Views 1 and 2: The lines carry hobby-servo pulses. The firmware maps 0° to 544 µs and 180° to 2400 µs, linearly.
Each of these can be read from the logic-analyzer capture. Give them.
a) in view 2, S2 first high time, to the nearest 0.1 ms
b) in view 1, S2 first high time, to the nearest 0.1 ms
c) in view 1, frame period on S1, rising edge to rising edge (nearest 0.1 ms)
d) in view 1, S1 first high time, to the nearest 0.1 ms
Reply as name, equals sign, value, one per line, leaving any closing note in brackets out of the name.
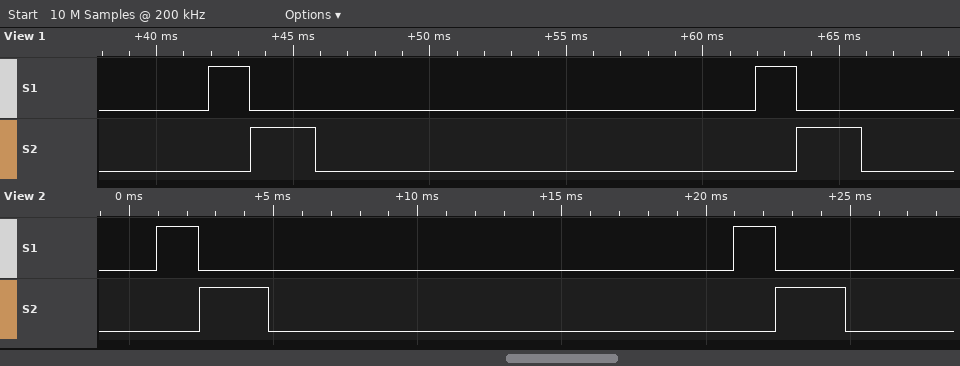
in view 2, S2 first high time, to the nearest 0.1 ms = 2.4 ms
in view 1, S2 first high time, to the nearest 0.1 ms = 2.4 ms
in view 1, frame period on S1, rising edge to rising edge = 20.0 ms
in view 1, S1 first high time, to the nearest 0.1 ms = 1.5 ms
